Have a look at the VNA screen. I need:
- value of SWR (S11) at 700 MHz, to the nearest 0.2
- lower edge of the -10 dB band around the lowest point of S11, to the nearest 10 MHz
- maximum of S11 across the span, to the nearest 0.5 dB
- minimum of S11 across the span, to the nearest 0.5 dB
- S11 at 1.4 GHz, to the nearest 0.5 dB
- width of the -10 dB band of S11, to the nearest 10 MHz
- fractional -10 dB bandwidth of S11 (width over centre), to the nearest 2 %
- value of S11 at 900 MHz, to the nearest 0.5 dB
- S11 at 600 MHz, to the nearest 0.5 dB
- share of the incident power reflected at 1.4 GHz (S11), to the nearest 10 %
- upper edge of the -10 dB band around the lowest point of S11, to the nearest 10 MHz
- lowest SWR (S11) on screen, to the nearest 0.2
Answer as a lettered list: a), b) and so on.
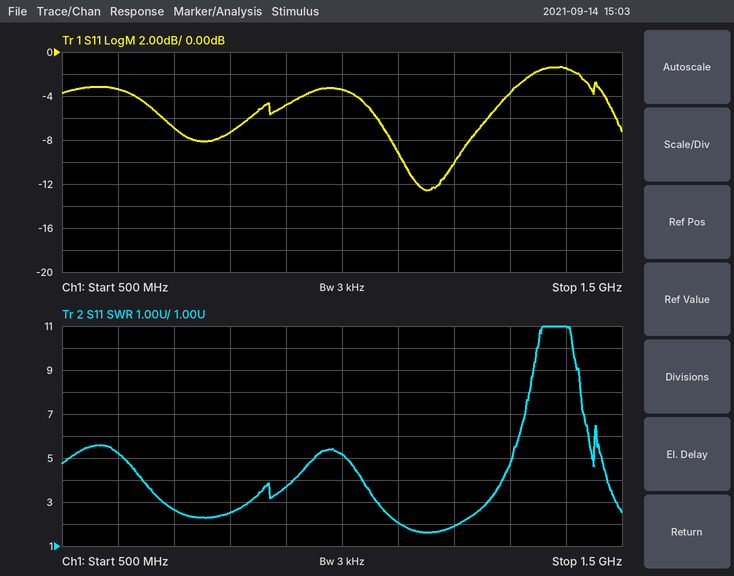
a) 2.6
b) 1.11 GHz
c) -1.5 dB
d) -12.5 dB
e) -1.5 dB
f) 90 MHz
g) 8 %
h) -5.0 dB
i) -3.5 dB
j) 70 %
k) 1.20 GHz
l) 1.6
